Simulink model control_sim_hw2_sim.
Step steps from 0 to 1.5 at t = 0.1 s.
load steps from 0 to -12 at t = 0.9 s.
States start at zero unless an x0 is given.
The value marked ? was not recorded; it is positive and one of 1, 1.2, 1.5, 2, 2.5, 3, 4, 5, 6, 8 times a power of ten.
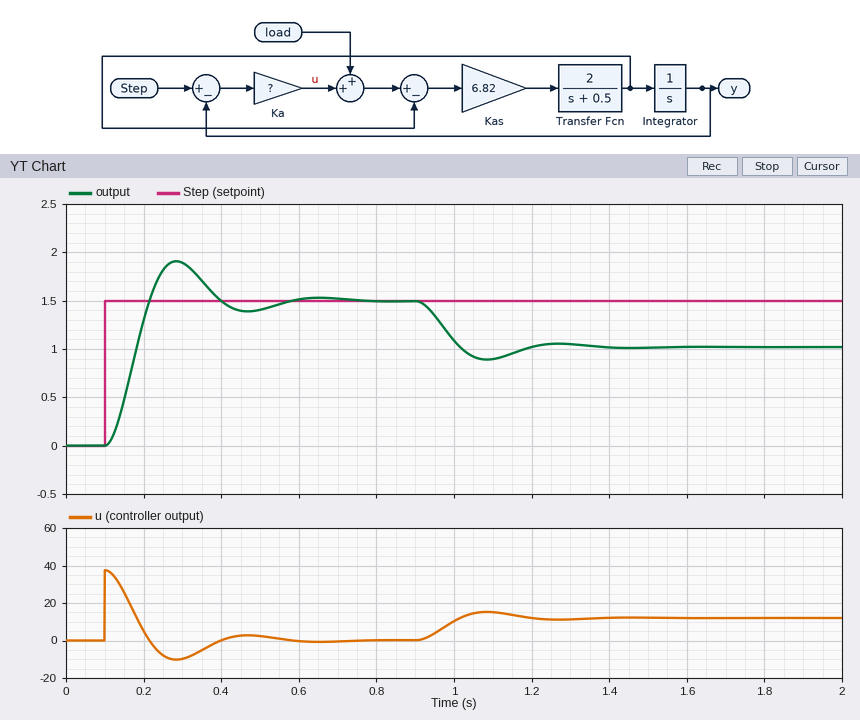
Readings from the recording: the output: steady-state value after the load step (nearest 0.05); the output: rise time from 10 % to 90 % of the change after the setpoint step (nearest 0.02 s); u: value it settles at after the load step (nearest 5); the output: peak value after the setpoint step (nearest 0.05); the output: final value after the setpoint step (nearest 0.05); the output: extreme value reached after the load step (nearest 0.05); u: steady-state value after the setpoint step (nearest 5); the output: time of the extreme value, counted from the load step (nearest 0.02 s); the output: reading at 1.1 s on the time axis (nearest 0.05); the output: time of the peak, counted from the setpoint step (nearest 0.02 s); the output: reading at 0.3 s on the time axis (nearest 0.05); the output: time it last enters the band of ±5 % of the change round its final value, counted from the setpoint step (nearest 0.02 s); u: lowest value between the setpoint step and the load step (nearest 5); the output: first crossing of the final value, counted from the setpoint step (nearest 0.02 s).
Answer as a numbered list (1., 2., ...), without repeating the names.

1. 1.00
2. 0.08 s
3. 10
4. 1.90
5. 1.50
6. 0.90
7. 0
8. 0.18 s
9. 0.90
10. 0.18 s
11. 1.90
12. 0.42 s
13. -10
14. 0.12 s
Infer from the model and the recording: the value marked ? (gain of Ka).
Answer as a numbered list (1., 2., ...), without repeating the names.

1. 25
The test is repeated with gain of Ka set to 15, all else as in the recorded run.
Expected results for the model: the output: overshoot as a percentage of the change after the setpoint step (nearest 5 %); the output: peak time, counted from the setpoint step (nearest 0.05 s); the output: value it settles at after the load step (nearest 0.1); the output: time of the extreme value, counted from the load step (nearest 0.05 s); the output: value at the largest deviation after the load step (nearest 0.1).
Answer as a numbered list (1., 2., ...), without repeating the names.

1. 15 %
2. 0.25 s
3. 0.7
4. 0.25 s
5. 0.6
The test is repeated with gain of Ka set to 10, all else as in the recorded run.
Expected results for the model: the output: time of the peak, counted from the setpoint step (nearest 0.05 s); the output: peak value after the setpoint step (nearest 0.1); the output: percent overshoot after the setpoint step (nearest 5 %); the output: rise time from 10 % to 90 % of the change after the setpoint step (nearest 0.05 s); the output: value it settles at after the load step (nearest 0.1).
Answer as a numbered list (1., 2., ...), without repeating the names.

1. 0.35 s
2. 1.6
3. 10 %
4. 0.15 s
5. 0.3
